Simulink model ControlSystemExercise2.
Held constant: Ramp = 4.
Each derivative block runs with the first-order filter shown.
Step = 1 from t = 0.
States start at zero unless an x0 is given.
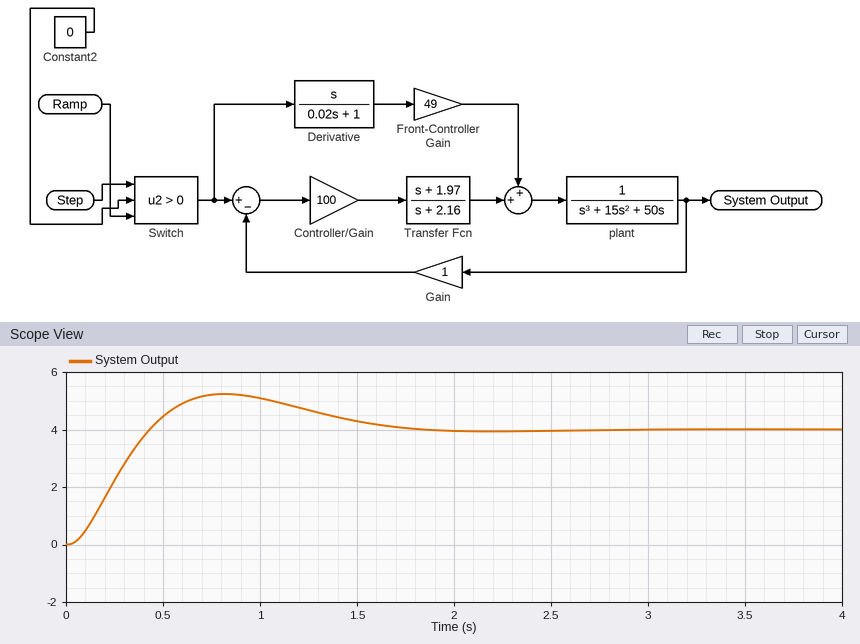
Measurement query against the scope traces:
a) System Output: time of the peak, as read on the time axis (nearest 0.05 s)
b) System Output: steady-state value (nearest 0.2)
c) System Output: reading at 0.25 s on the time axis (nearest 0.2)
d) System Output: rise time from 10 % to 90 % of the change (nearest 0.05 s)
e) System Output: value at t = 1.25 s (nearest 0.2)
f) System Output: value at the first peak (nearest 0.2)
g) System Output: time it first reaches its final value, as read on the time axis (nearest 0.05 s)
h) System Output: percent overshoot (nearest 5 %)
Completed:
0.80 s
4.0
2.2
0.30 s
4.6
5.2
0.45 s
30 %
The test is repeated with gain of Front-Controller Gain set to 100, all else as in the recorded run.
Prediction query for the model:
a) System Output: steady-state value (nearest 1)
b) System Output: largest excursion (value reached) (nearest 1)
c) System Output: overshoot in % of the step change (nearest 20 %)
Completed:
4
8
100 %
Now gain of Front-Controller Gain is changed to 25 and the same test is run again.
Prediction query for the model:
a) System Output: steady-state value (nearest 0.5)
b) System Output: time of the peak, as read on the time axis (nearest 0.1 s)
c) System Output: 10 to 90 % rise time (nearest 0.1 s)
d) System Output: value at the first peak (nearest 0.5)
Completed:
4.0
1.1 s
0.5 s
4.5
